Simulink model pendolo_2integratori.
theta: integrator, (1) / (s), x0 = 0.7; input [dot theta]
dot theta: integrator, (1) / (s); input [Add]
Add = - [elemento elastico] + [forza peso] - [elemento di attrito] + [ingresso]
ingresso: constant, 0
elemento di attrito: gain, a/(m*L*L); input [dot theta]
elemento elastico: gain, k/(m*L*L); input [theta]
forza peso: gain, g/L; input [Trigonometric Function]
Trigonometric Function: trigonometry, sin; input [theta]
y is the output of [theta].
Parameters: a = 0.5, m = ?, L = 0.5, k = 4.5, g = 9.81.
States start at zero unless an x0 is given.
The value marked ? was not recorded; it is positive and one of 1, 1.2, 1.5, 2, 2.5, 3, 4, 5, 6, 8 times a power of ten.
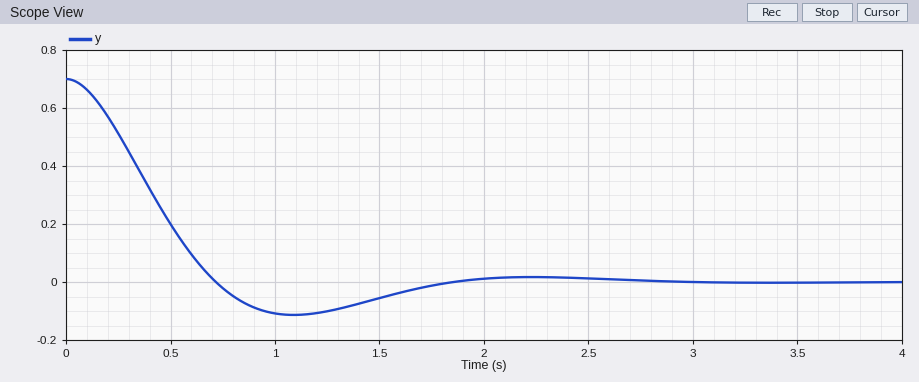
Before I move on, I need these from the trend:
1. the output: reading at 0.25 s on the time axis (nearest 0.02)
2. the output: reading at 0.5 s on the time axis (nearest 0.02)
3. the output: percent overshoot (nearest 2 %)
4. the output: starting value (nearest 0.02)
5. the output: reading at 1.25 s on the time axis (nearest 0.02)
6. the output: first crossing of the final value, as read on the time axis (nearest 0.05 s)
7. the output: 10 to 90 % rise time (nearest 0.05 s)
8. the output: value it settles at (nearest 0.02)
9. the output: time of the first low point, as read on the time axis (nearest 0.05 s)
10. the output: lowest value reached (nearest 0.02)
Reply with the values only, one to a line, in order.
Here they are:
0.52
0.20
16 %
0.70
-0.10
0.70 s
0.50 s
0.00
1.10 s
-0.12
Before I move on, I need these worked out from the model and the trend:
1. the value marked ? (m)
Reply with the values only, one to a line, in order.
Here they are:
0.6
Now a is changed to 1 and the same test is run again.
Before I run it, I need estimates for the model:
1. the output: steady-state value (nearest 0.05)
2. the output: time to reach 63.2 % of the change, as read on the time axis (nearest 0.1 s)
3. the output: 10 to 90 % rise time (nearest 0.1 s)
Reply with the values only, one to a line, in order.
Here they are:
0.00
0.6 s
1.0 s
